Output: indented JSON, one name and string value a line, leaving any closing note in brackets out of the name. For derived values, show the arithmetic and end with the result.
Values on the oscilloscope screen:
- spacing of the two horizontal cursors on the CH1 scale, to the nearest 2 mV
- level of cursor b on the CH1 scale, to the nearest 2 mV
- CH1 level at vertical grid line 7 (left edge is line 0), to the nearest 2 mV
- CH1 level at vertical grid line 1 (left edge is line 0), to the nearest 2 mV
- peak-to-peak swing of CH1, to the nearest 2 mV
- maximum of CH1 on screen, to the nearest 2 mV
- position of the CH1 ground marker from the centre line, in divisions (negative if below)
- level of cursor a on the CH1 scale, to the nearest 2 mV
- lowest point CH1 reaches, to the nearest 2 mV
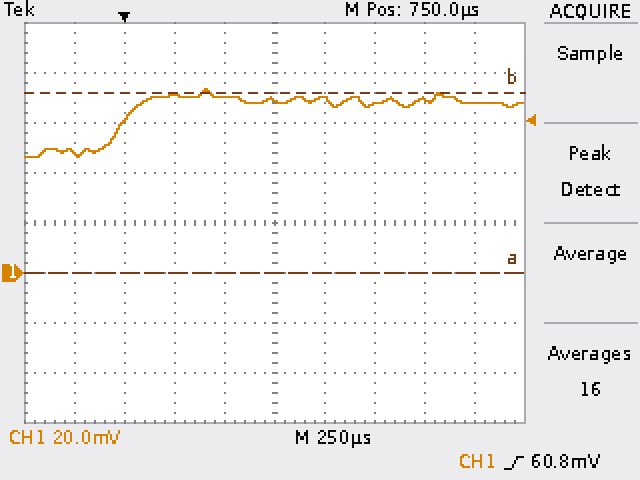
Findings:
{
  "spacing of the two horizontal cursors on the CH1 scale, to the nearest 2 mV": "72 mV",
  "level of cursor b on the CH1 scale, to the nearest 2 mV": "72 mV",
  "CH1 level at vertical grid line 7 (left edge is line 0), to the nearest 2 mV": "68 mV",
  "CH1 level at vertical grid line 1 (left edge is line 0), to the nearest 2 mV": "48 mV",
  "peak-to-peak swing of CH1, to the nearest 2 mV": "74 mV − (46 mV) = 28 mV",
  "maximum of CH1 on screen, to the nearest 2 mV": "74 mV",
  "position of the CH1 ground marker from the centre line, in divisions": "-1.0 div",
  "level of cursor a on the CH1 scale, to the nearest 2 mV": "0 mV",
  "lowest point CH1 reaches, to the nearest 2 mV": "46 mV"
}
